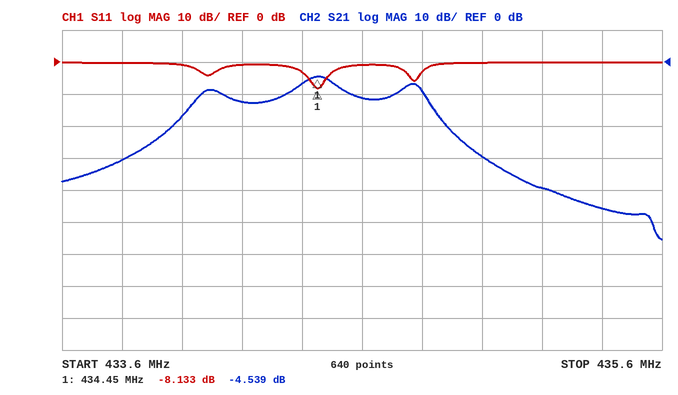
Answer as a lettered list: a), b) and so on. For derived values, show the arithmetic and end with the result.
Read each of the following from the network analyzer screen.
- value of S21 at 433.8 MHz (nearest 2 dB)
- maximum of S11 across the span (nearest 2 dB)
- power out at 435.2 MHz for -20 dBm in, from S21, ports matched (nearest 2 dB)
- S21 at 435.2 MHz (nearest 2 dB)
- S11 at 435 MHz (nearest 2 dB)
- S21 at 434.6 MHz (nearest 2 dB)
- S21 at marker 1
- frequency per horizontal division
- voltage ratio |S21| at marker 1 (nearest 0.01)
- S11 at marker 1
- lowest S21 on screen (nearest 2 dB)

a) -30 dB
b) 0 dB
c) -20 dBm + (-40 dB) = -60 dBm
d) -40 dB
e) 0 dB
f) -12 dB
g) -4.539 dB
h) 200 kHz
i) 10^(-4.539/20) ≈ 0.59
j) -8.133 dB
k) -56 dB
